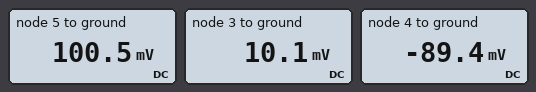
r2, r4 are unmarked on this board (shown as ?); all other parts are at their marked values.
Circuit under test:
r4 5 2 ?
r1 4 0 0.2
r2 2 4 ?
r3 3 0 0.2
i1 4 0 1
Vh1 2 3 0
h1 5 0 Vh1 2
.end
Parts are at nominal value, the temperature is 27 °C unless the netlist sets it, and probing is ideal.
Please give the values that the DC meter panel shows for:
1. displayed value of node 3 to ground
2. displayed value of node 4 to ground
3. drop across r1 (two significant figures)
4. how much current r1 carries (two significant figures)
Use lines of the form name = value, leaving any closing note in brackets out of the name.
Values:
displayed value of node 3 to ground = 10.1 mV
displayed value of node 4 to ground = -89.4 mV
drop across r1 = 89 mV
how much current r1 carries = 450 mA
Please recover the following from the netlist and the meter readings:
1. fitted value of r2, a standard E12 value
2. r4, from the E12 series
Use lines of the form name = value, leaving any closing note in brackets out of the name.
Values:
fitted value of r2, a standard E12 value = 0.18 Ω
r4, from the E12 series = 0.15 Ω
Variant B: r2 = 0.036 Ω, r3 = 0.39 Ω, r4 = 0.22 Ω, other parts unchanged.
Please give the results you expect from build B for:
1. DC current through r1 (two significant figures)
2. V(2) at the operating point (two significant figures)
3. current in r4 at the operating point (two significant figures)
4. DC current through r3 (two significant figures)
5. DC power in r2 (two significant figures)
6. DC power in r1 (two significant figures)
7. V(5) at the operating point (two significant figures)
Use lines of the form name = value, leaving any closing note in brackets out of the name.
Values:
DC current through r1 = 150 mA
V(2) at the operating point = 71 mV
current in r4 at the operating point = 1.3 A
DC current through r3 = 180 mA
DC power in r2 = 47 mW
DC power in r1 = 4.4 mW
V(5) at the operating point = 360 mV
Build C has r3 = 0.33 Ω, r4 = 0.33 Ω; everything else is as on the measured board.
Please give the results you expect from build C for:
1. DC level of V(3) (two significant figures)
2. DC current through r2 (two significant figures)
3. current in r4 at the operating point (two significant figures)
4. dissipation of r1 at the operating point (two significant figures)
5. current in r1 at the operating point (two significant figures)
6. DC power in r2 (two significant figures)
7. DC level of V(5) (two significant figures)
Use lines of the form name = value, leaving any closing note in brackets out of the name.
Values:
DC level of V(3) = 54 mV
DC current through r2 = 670 mA
current in r4 at the operating point = 830 mA
dissipation of r1 at the operating point = 22 mW
current in r1 at the operating point = 330 mA
DC power in r2 = 81 mW
DC level of V(5) = 330 mV
